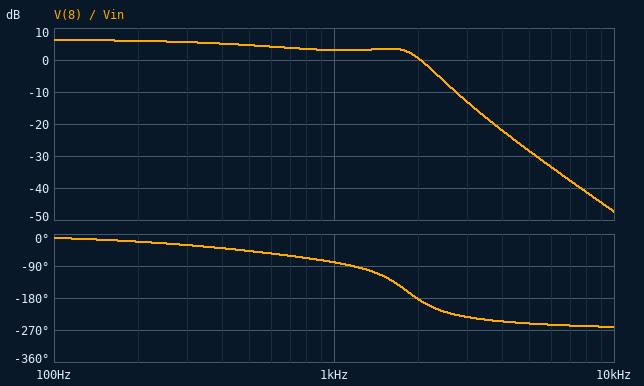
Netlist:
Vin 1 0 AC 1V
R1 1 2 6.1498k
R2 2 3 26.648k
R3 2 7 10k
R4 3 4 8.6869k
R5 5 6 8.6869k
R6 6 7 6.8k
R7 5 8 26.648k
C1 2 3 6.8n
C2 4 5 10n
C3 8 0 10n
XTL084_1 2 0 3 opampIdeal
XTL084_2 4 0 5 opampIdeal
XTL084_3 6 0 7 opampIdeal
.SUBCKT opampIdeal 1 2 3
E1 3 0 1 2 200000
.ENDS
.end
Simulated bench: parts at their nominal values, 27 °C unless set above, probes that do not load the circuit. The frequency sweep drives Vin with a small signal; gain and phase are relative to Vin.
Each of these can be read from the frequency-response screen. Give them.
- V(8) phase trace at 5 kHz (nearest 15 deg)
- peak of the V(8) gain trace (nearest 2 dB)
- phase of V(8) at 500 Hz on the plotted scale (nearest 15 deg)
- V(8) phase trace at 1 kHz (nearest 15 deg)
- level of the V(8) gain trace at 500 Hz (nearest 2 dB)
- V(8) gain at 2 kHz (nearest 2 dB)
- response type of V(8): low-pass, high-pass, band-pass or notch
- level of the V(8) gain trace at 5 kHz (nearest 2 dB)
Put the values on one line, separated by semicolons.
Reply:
-255 deg; 6 dB; -45 deg; -75 deg; 4 dB; 0 dB; low-pass; -28 dB
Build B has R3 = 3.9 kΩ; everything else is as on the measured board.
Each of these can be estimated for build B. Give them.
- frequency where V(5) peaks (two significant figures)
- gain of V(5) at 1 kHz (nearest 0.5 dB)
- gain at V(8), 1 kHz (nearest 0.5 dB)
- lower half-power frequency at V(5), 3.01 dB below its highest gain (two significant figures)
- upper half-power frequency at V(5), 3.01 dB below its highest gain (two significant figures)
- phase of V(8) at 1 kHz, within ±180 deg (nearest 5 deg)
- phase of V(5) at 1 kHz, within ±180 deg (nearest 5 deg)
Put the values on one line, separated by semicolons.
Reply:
2.9 kHz; -1.0 dB; -6.5 dB; 2.4 kHz; 3.3 kHz; -65 deg; -5 deg
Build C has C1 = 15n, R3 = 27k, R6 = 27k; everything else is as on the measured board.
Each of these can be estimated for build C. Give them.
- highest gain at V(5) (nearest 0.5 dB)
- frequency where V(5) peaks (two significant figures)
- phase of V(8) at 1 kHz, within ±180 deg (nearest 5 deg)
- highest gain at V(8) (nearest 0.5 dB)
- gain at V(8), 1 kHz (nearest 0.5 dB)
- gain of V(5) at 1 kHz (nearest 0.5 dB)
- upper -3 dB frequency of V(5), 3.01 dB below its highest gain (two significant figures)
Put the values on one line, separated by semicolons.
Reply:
14.5 dB; 1.5 kHz; -75 deg; 6.0 dB; 2.0 dB; 7.5 dB; 1.7 kHz
